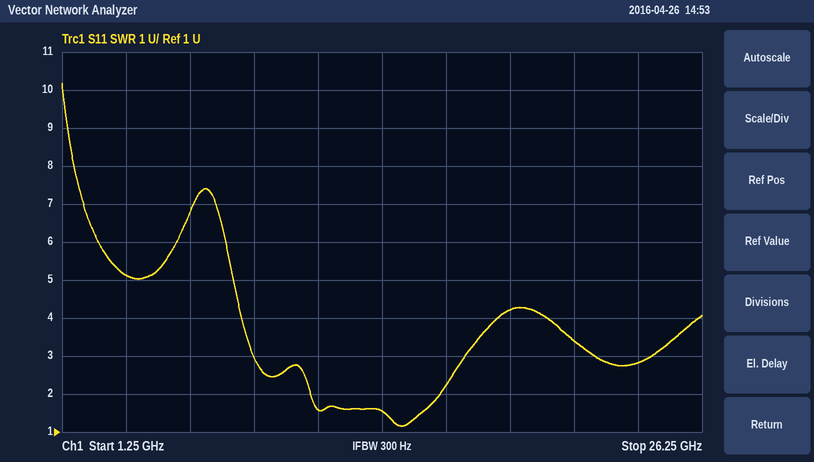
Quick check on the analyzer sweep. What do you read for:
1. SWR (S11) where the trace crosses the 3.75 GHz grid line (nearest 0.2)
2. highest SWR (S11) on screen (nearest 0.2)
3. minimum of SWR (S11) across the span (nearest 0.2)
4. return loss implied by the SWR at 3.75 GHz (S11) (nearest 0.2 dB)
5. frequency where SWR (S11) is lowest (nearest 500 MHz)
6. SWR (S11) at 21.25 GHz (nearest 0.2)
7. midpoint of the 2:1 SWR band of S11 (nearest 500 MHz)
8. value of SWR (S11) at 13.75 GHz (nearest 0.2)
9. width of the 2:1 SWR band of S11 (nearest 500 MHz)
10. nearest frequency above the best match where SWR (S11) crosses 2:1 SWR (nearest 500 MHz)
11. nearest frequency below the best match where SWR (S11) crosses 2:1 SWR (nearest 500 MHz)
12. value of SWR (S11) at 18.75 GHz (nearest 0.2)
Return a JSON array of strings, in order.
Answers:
["5.2", "10.2", "1.2", "3.4 dB", "14.5 GHz", "3.4", "13.5 GHz", "1.6", "5.0 GHz", "16.0 GHz", "11.0 GHz", "4.2"]
